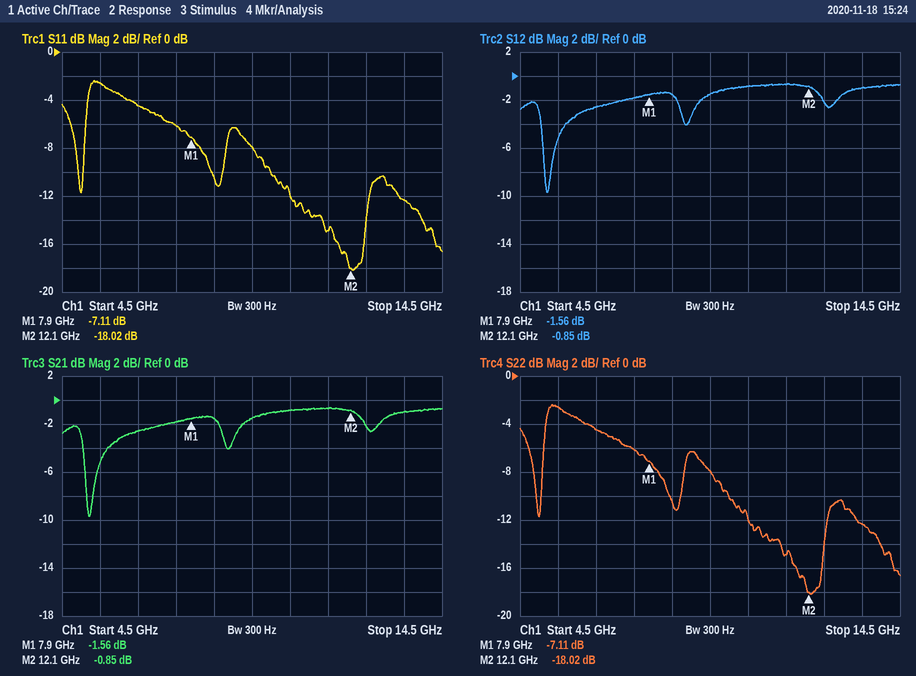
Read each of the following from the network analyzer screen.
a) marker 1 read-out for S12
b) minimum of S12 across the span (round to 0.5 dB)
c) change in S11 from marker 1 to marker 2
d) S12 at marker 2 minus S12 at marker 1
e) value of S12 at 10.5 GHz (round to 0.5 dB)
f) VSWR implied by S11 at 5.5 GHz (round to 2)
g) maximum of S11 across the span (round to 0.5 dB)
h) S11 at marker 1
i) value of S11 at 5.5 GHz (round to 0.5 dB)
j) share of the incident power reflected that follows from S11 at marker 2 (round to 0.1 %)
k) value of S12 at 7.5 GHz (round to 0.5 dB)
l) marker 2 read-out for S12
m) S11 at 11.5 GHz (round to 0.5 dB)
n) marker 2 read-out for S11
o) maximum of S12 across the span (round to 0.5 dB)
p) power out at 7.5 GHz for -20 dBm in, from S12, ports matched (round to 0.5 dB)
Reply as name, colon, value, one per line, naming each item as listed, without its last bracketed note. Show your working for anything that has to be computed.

marker 1 read-out for S12: -1.56 dB
minimum of S12 across the span: -9.5 dB
change in S11 from marker 1 to marker 2: -18.02 − (-7.11) = -10.91 dB
S12 at marker 2 minus S12 at marker 1: -0.85 − (-1.56) = 0.71 dB
value of S12 at 10.5 GHz: -1.0 dB
VSWR implied by S11 at 5.5 GHz: |Γ| = 10^(-2.5/20) = 0.7499; VSWR = (1 + 0.7499)/(1 − 0.7499) ≈ 7.00, so 6 to the nearest 2
maximum of S11 across the span: -2.5 dB
S11 at marker 1: -7.11 dB
value of S11 at 5.5 GHz: -2.5 dB
share of the incident power reflected that follows from S11 at marker 2: 10^(-18.02/10) ≈ 1.6 %
value of S12 at 7.5 GHz: -2.0 dB
marker 2 read-out for S12: -0.85 dB
S11 at 11.5 GHz: -15.0 dB
marker 2 read-out for S11: -18.02 dB
maximum of S12 across the span: -0.5 dB
power out at 7.5 GHz for -20 dBm in, from S12, ports matched: -20 dBm + (-2.0 dB) = -22.0 dBm
